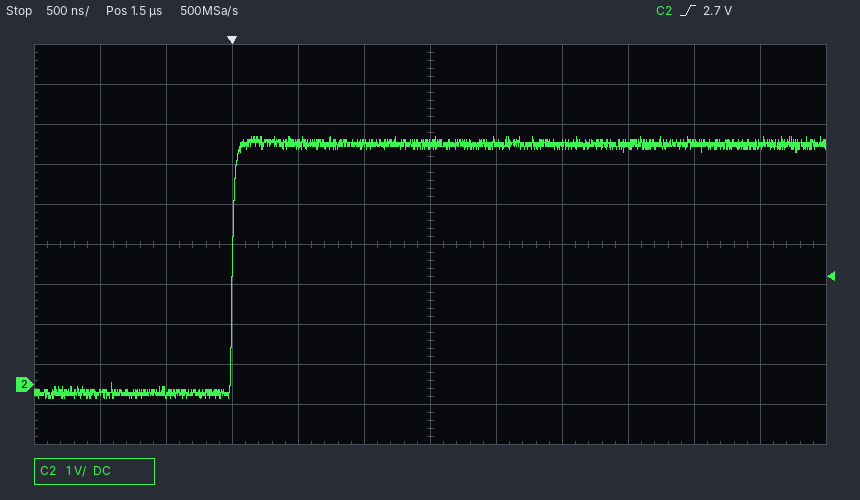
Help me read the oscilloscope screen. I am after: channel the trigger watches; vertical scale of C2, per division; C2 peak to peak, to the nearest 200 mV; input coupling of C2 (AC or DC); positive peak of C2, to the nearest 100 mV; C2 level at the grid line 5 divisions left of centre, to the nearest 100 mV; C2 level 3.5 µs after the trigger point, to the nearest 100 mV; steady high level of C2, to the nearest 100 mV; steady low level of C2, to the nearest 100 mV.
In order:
C2
1 V
6.6 V
DC
6.2 V
-200 mV
6.0 V
6.0 V
-200 mV
